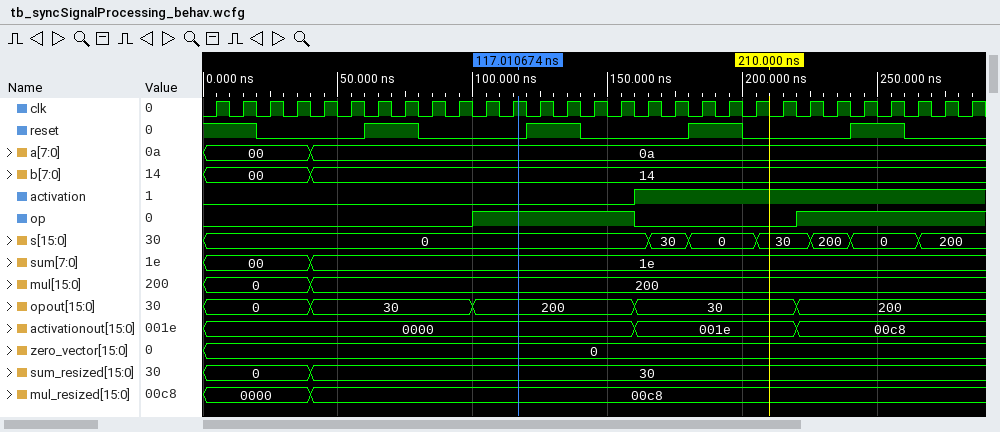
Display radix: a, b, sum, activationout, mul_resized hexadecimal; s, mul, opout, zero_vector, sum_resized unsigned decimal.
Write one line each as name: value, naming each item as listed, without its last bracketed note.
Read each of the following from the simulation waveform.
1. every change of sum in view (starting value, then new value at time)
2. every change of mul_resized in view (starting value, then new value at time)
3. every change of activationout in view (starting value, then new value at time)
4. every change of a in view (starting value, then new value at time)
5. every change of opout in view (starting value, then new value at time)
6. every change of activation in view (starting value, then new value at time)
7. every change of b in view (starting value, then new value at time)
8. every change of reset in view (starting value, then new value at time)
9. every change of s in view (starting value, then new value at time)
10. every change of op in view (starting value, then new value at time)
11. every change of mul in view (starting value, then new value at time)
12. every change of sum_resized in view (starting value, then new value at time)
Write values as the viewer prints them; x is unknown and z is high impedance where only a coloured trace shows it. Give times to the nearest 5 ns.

every change of sum in view: 00, 1e at 40 ns
every change of mul_resized in view: 0000, 00c8 at 40 ns
every change of activationout in view: 0000, 001e at 160 ns, 00c8 at 220 ns
every change of a in view: 00, 0a at 40 ns
every change of opout in view: 0, 30 at 40 ns, 200 at 100 ns, 30 at 160 ns, 200 at 220 ns
every change of activation in view: 0, 1 at 160 ns
every change of b in view: 00, 14 at 40 ns
every change of reset in view: 1, 0 at 20 ns, 1 at 60 ns, 0 at 80 ns, 1 at 120 ns, 0 at 140 ns, 1 at 180 ns, 0 at 200 ns, 1 at 240 ns, 0 at 260 ns
every change of s in view: 0, 30 at 165 ns, 0 at 180 ns, 30 at 205 ns, 200 at 225 ns, 0 at 240 ns, 200 at 265 ns
every change of op in view: 0, 1 at 100 ns, 0 at 160 ns, 1 at 220 ns
every change of mul in view: 0, 200 at 40 ns
every change of sum_resized in view: 0, 30 at 40 ns
